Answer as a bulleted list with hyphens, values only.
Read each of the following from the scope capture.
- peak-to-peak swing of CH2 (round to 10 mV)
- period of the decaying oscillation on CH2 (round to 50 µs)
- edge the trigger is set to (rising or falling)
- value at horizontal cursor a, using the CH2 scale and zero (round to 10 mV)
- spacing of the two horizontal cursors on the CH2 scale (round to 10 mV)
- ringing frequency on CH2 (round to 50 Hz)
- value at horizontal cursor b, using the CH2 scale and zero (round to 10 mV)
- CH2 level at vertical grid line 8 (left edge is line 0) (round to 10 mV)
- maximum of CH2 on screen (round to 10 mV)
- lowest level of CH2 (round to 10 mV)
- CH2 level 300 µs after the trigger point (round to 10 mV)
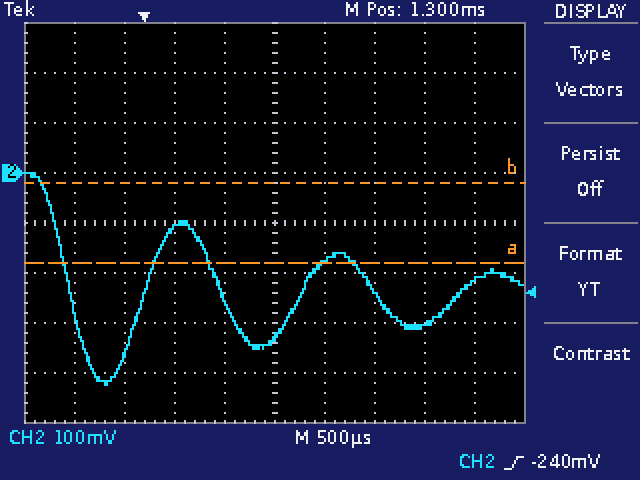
- 420 mV
- 1.55 ms
- rising
- -180 mV
- 160 mV
- 650 Hz
- -20 mV
- -300 mV
- 0 mV
- -420 mV
- -110 mV
